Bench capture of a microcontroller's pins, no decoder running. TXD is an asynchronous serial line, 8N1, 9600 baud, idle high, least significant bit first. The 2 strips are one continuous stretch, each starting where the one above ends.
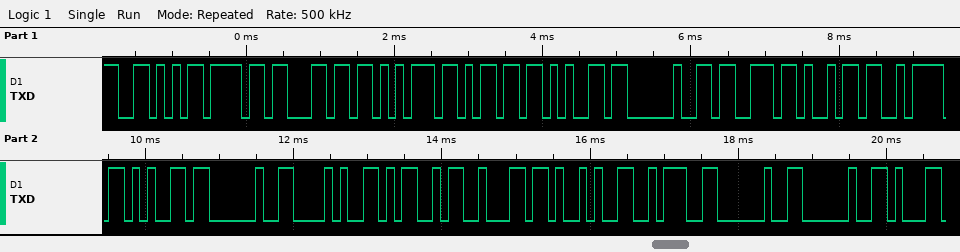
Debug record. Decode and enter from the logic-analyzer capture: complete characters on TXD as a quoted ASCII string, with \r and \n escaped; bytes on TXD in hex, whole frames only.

"Volume size (Mb):  "
56 6F 6C 75 6D 65 20 73 69 7A 65 20 28 4D 62 29 3A 20 20
